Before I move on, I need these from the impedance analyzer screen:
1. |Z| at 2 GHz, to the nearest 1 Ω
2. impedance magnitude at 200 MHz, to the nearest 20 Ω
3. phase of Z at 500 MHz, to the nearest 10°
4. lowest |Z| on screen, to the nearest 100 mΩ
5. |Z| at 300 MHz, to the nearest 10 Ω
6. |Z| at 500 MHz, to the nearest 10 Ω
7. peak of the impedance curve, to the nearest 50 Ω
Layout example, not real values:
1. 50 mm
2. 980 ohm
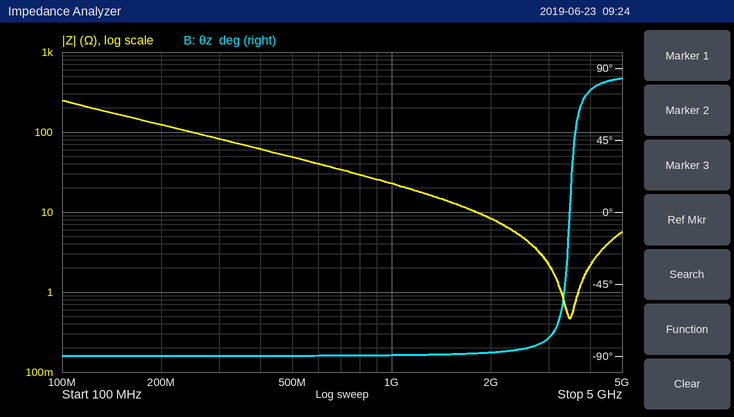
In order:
1. 8 Ω
2. 120 Ω
3. -90°
4. 500 mΩ
5. 80 Ω
6. 50 Ω
7. 250 Ω
